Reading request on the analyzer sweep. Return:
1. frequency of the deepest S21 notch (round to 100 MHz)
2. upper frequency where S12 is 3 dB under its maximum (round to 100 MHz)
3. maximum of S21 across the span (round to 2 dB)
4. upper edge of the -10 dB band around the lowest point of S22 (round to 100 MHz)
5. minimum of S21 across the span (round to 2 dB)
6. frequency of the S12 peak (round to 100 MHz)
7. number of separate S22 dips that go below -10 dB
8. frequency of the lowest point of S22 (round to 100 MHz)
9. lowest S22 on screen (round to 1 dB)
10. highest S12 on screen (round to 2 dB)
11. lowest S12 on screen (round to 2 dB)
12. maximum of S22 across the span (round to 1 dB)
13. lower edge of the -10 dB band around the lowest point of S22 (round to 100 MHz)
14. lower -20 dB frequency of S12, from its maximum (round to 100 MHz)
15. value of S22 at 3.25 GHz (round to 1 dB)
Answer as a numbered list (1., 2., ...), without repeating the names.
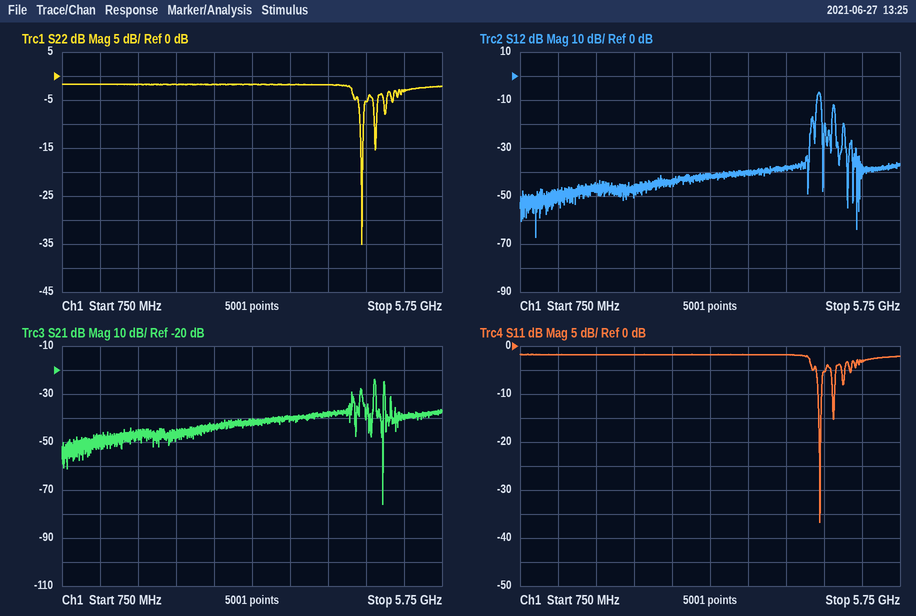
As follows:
1. 5.0 GHz
2. 4.7 GHz
3. -24 dB
4. 4.7 GHz
5. -76 dB
6. 4.7 GHz
7. 2
8. 4.7 GHz
9. -35 dB
10. -6 dB
11. -68 dB
12. -2 dB
13. 4.7 GHz
14. 4.6 GHz
15. -2 dB
